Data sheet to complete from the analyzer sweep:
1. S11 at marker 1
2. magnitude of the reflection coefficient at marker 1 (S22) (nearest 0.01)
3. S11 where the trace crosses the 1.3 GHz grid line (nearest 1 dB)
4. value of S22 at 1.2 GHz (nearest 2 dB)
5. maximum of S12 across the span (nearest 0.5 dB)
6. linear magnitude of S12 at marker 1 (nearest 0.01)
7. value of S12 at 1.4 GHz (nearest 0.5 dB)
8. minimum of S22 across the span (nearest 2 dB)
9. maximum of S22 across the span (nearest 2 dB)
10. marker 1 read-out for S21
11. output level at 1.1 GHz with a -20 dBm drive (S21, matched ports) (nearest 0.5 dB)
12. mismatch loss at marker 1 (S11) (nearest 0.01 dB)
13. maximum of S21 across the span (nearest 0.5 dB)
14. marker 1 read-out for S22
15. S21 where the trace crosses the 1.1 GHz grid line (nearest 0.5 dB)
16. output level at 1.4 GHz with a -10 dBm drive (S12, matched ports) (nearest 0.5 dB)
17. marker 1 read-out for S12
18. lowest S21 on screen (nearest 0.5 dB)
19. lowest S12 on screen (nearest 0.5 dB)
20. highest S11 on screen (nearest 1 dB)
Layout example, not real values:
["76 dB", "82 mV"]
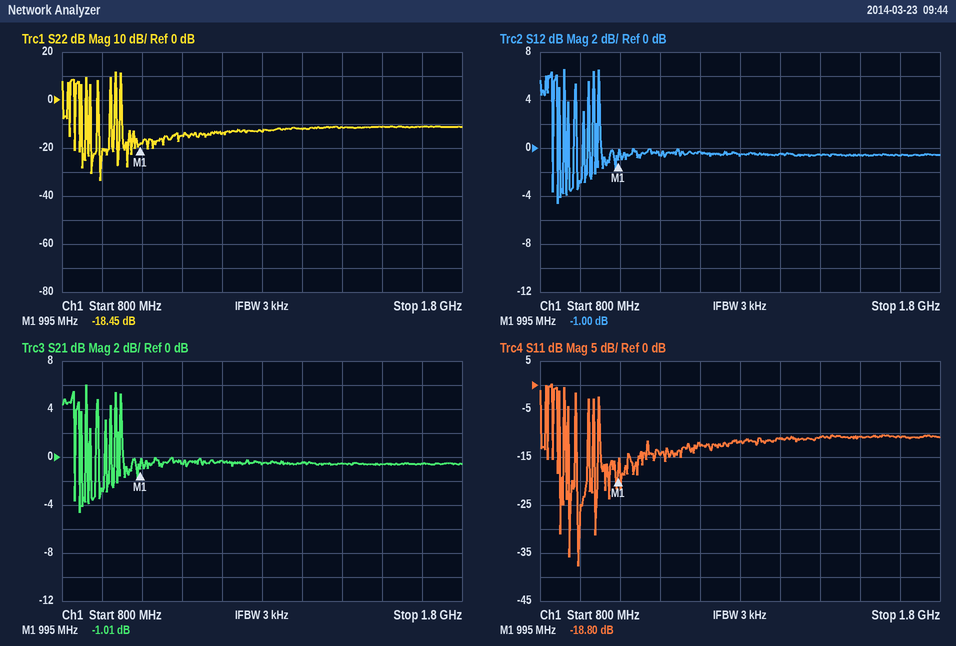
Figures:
["-18.80 dB", "0.12", "-12 dB", "-14 dB", "6.5 dB", "0.89", "-0.5 dB", "-34 dB", "12 dB", "-1.01 dB", "-20.5 dBm", "0.06 dB", "6.0 dB", "-18.45 dB", "-0.5 dB", "-10.5 dBm", "-1.00 dB", "-4.5 dB", "-4.5 dB", "0 dB"]
